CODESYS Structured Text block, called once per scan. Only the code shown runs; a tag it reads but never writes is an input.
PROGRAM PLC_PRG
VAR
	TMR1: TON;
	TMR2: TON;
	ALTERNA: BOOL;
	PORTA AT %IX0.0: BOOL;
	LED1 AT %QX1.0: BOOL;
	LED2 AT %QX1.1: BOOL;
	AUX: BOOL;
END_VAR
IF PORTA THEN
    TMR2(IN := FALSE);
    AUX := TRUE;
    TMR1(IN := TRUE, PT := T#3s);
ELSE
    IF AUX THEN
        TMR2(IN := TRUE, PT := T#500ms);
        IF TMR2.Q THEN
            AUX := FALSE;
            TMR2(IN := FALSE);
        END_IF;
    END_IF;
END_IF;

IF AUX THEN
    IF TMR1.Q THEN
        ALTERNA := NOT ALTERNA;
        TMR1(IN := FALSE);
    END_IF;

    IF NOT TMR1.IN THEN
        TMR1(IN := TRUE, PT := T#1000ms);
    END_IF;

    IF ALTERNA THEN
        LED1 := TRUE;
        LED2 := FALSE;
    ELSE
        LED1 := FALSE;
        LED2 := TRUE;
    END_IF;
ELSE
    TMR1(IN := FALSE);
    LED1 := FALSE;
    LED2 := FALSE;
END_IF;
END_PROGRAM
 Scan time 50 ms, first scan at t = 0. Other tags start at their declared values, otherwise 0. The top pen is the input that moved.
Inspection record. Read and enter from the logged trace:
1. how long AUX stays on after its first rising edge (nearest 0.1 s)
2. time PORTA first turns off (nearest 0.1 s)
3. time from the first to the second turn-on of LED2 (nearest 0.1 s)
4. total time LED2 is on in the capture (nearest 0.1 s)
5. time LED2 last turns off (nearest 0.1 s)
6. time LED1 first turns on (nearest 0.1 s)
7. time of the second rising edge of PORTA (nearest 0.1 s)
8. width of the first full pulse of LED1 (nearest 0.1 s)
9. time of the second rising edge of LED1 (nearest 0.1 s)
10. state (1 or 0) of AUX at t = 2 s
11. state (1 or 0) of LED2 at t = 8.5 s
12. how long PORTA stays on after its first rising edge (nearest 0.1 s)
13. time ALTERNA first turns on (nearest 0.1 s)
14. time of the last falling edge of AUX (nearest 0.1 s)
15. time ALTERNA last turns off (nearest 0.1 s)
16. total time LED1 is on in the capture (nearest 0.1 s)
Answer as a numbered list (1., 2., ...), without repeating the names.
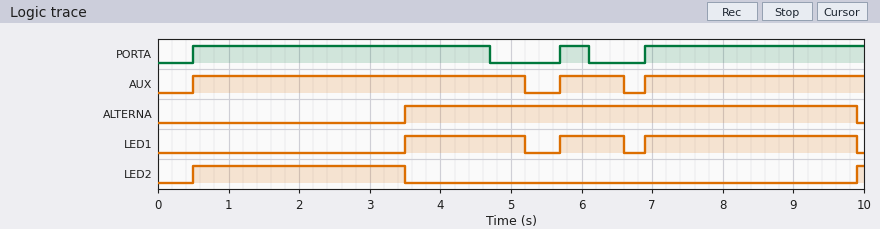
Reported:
1. 4.7 s
2. 4.7 s
3. 9.4 s
4. 3.1 s
5. 3.5 s
6. 3.5 s
7. 5.7 s
8. 1.7 s
9. 5.7 s
10. 1
11. 0
12. 4.2 s
13. 3.5 s
14. 6.6 s
15. 9.9 s
16. 5.6 s
